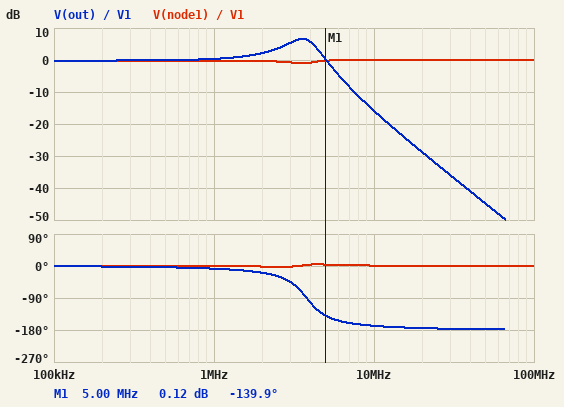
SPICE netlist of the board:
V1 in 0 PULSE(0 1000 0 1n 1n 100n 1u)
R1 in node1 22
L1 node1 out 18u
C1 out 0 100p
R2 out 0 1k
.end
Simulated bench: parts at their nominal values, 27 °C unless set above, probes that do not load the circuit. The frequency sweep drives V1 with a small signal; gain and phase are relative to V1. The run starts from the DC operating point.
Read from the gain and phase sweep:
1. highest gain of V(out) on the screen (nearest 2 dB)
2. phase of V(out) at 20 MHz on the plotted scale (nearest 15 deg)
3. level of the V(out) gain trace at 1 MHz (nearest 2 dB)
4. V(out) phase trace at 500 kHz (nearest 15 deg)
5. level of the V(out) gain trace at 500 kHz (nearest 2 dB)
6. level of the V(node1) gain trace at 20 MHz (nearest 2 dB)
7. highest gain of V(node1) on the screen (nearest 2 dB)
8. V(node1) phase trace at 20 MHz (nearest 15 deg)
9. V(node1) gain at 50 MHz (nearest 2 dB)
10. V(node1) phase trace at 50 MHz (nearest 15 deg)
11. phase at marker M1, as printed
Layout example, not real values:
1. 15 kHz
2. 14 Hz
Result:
1. 6 dB
2. -180 deg
3. 0 dB
4. 0 deg
5. 0 dB
6. 0 dB
7. 0 dB
8. 0 deg
9. 0 dB
10. 0 deg
11. -139.9 deg
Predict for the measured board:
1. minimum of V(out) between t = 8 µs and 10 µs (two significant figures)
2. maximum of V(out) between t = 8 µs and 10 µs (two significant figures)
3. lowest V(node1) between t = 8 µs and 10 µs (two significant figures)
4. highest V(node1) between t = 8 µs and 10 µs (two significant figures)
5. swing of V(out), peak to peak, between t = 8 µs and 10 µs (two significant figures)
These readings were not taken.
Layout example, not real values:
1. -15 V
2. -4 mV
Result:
1. -620 V
2. 1.3 kV
3. -49 V
4. 1.0 kV
5. 1.9 kV
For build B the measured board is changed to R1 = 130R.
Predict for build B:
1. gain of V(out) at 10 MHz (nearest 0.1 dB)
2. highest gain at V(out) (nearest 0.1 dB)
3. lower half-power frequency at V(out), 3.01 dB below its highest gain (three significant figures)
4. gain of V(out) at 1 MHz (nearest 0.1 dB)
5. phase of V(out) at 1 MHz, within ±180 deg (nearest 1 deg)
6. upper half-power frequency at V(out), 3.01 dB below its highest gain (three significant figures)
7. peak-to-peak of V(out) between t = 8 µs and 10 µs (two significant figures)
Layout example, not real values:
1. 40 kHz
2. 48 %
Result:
1. -16.0 dB
2. 2.7 dB
3. 1.37 MHz
4. -0.6 dB
5. -10 deg
6. 4.73 MHz
7. 1.4 kV
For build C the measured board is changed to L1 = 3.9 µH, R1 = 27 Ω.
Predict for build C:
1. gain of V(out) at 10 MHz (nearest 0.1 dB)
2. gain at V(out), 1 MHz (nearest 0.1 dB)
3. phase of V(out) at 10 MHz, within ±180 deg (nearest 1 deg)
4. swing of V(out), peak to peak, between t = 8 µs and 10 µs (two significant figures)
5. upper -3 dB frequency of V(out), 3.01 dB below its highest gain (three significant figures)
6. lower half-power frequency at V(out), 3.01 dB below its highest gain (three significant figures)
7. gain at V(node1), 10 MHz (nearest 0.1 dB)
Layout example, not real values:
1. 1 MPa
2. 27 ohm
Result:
1. 3.6 dB
2. -0.1 dB
3. -141 deg
4. 2.1 kV
5. 9.21 MHz
6. 6.43 MHz
7. -0.9 dB
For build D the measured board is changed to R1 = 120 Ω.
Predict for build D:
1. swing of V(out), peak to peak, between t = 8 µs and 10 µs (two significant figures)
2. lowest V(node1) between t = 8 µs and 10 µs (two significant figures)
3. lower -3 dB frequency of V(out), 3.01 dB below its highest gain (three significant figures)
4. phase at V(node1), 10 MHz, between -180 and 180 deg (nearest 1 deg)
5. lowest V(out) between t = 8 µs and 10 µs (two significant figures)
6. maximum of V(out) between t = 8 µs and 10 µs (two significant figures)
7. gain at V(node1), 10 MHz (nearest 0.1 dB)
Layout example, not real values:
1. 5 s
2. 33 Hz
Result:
1. 1.5 kV
2. -210 V
3. 1.52 MHz
4. 7 deg
5. -360 V
6. 1.1 kV
7. -0.1 dB
